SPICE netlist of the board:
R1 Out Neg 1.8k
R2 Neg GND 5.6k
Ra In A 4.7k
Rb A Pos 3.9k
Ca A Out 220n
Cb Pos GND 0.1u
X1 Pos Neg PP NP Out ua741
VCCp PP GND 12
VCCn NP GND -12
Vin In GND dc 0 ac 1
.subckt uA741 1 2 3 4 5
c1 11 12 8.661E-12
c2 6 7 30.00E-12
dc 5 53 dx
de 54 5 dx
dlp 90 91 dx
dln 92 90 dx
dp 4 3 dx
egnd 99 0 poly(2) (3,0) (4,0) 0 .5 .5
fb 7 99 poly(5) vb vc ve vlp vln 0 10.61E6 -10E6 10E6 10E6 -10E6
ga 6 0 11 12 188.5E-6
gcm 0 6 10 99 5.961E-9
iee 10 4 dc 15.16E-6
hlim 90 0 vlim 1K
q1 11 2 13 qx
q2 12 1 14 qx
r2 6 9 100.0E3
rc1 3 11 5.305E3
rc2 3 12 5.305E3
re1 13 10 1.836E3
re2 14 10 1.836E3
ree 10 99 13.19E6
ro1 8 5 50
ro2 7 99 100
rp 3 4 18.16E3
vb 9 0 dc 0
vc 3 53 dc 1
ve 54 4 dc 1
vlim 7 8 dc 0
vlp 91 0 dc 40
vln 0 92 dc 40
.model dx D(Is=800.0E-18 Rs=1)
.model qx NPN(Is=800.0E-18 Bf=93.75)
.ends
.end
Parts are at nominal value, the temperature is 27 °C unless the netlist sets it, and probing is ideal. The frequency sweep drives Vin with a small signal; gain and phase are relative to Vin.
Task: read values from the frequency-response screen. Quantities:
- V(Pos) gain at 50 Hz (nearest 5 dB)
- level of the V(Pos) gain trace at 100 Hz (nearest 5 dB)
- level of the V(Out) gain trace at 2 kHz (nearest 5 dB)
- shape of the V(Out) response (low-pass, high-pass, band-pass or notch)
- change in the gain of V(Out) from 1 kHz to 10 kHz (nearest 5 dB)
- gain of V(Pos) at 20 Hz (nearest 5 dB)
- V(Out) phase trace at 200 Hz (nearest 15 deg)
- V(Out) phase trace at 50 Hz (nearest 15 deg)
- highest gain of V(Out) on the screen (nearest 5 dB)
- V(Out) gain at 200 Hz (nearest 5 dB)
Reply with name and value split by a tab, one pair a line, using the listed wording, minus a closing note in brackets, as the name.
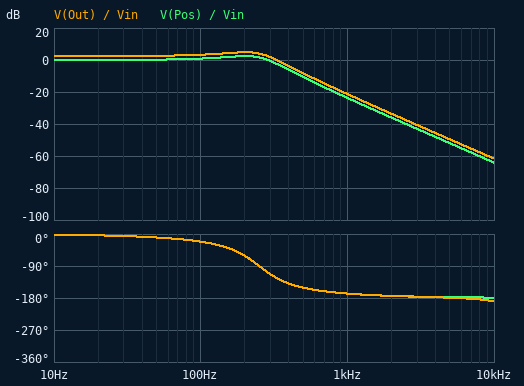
V(Pos) gain at 50 Hz	0 dB
level of the V(Pos) gain trace at 100 Hz	0 dB
level of the V(Out) gain trace at 2 kHz	-35 dB
shape of the V(Out) response	low-pass
change in the gain of V(Out) from 1 kHz to 10 kHz	-40 dB
gain of V(Pos) at 20 Hz	0 dB
V(Out) phase trace at 200 Hz	-60 deg
V(Out) phase trace at 50 Hz	-15 deg
highest gain of V(Out) on the screen	5 dB
V(Out) gain at 200 Hz	5 dB
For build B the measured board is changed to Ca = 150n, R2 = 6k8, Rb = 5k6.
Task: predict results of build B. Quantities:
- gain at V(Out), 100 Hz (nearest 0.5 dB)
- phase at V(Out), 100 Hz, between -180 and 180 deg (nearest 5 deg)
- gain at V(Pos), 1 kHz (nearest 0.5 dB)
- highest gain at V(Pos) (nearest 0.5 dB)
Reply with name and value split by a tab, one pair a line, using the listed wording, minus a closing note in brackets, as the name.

gain at V(Out), 100 Hz	2.0 dB
phase at V(Out), 100 Hz, between -180 and 180 deg	-30 deg
gain at V(Pos), 1 kHz	-24.0 dB
highest gain at V(Pos)	0 dB
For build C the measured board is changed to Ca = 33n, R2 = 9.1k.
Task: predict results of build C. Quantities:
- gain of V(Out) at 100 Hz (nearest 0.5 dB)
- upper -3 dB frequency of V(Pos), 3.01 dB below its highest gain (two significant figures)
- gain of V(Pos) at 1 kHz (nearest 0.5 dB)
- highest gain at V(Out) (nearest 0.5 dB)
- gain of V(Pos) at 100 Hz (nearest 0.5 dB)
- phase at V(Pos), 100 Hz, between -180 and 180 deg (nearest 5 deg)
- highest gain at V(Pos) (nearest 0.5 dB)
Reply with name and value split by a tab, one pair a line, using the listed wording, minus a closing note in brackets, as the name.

gain of V(Out) at 100 Hz	0.5 dB
upper -3 dB frequency of V(Pos), 3.01 dB below its highest gain	210 Hz
gain of V(Pos) at 1 kHz	-14.5 dB
highest gain at V(Out)	1.5 dB
gain of V(Pos) at 100 Hz	-1.0 dB
phase at V(Pos), 100 Hz, between -180 and 180 deg	-30 deg
highest gain at V(Pos)	0 dB
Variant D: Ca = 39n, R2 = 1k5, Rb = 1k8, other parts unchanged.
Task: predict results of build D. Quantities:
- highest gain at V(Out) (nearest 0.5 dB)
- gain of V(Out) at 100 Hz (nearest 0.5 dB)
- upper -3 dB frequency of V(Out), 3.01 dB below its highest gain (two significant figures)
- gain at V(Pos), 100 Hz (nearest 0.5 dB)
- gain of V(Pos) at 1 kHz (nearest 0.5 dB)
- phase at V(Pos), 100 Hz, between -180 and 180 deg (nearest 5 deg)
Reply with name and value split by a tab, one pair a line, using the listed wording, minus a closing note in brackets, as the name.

highest gain at V(Out)	7.0 dB
gain of V(Out) at 100 Hz	6.5 dB
upper -3 dB frequency of V(Out), 3.01 dB below its highest gain	450 Hz
gain at V(Pos), 100 Hz	0 dB
gain of V(Pos) at 1 kHz	-8.5 dB
phase at V(Pos), 100 Hz, between -180 and 180 deg	-15 deg
